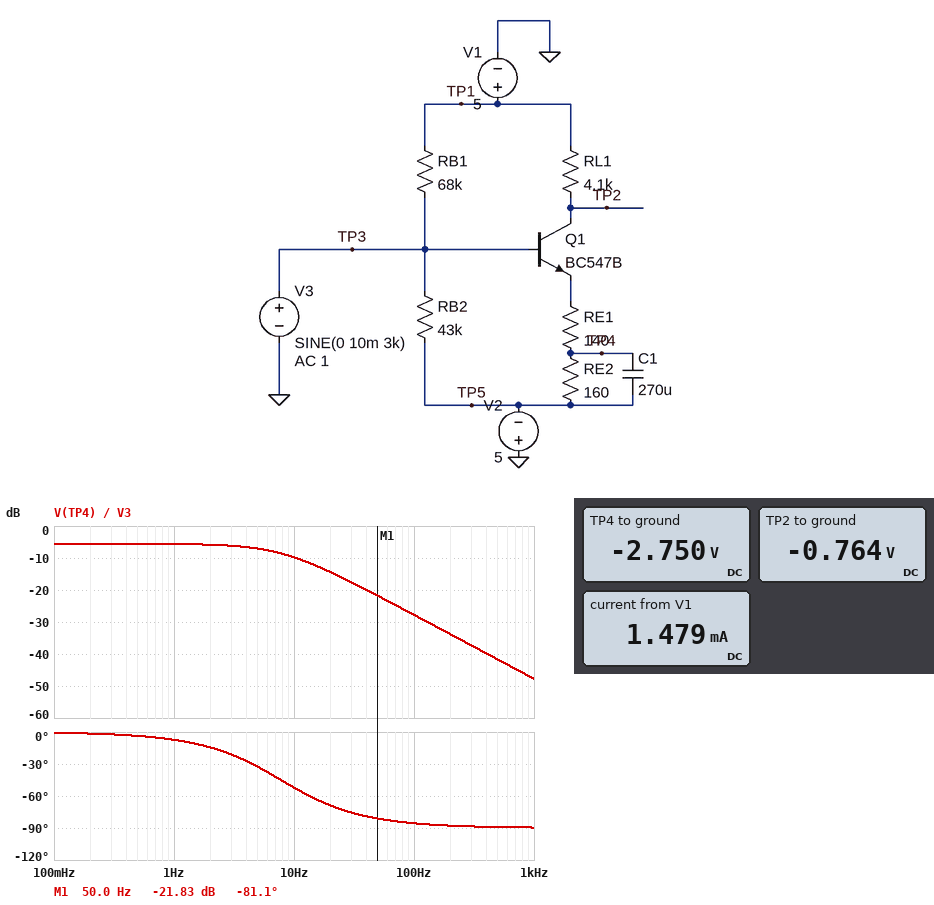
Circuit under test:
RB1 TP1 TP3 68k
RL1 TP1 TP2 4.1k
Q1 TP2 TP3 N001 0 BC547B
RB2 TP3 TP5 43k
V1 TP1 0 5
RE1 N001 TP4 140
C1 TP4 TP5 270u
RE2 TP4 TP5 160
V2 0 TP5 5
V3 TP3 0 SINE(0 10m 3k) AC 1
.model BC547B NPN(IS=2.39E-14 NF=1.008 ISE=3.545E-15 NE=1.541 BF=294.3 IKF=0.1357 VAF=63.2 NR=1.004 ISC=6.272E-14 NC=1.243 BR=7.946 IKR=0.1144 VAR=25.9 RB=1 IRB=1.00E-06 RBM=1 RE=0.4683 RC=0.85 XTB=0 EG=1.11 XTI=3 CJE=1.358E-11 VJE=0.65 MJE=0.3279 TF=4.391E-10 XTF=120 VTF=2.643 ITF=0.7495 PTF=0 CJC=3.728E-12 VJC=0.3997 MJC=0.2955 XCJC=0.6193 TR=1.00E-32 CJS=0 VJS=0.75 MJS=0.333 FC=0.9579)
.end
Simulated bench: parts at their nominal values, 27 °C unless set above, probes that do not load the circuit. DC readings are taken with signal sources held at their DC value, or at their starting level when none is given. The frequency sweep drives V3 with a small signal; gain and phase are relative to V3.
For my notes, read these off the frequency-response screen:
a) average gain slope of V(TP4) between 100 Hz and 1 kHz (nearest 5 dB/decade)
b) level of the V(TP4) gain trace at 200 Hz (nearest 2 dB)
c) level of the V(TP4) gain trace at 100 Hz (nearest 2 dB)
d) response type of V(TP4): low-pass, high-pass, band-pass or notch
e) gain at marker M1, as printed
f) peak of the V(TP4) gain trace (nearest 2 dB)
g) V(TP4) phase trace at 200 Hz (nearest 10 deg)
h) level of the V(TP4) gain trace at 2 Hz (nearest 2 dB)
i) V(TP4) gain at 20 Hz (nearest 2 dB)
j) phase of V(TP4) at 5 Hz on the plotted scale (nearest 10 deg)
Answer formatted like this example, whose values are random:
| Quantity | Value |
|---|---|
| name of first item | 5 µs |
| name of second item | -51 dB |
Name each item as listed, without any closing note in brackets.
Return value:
| Quantity | Value |
|---|---|
| average gain slope of V(TP4) between 100 Hz and 1 kHz | -20 dB/decade |
| level of the V(TP4) gain trace at 200 Hz | -34 dB |
| level of the V(TP4) gain trace at 100 Hz | -28 dB |
| response type of V(TP4): low-pass, high-pass, band-pass or notch | low-pass |
| gain at marker M1, as printed | -21.83 dB |
| peak of the V(TP4) gain trace | -6 dB |
| V(TP4) phase trace at 200 Hz | -90 deg |
| level of the V(TP4) gain trace at 2 Hz | -6 dB |
| V(TP4) gain at 20 Hz | -14 dB |
| phase of V(TP4) at 5 Hz on the plotted scale | -30 deg |
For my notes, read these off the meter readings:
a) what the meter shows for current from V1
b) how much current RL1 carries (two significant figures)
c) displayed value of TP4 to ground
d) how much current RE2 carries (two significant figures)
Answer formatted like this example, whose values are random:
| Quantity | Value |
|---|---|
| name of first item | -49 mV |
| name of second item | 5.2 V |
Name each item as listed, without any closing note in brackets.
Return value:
| Quantity | Value |
|---|---|
| what the meter shows for current from V1 | 1.479 mA |
| how much current RL1 carries | 1.4 mA |
| displayed value of TP4 to ground | -2.750 V |
| how much current RE2 carries | 14 mA |
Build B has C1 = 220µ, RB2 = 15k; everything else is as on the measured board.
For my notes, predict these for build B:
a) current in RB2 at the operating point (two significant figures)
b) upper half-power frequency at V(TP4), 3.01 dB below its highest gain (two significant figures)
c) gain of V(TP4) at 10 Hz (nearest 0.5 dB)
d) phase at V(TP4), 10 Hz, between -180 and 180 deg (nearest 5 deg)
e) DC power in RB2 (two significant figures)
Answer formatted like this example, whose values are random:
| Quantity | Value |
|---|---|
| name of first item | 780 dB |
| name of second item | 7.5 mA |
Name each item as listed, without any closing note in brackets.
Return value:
| Quantity | Value |
|---|---|
| current in RB2 at the operating point | 330 µA |
| upper half-power frequency at V(TP4), 3.01 dB below its highest gain | 9.6 Hz |
| gain of V(TP4) at 10 Hz | -9.0 dB |
| phase at V(TP4), 10 Hz, between -180 and 180 deg | -45 deg |
| DC power in RB2 | 1.7 mW |
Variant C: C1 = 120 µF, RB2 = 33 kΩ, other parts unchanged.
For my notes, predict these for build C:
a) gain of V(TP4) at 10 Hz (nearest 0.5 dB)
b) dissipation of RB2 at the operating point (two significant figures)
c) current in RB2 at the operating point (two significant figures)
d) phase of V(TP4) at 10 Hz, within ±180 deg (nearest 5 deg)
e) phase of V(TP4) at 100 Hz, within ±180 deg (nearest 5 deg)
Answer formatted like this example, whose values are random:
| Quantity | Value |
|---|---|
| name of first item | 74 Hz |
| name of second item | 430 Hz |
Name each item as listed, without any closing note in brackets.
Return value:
| Quantity | Value |
|---|---|
| gain of V(TP4) at 10 Hz | -7.0 dB |
| dissipation of RB2 at the operating point | 760 µW |
| current in RB2 at the operating point | 150 µA |
| phase of V(TP4) at 10 Hz, within ±180 deg | -30 deg |
| phase of V(TP4) at 100 Hz, within ±180 deg | -80 deg |
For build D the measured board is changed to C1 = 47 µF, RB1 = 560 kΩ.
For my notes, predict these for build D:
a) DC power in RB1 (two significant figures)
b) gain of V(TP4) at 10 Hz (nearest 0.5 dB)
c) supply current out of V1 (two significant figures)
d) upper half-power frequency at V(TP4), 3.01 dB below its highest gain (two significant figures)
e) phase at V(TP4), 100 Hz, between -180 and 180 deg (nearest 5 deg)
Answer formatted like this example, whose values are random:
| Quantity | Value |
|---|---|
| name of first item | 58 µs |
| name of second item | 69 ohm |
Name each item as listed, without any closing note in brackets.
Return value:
| Quantity | Value |
|---|---|
| DC power in RB1 | 45 µW |
| gain of V(TP4) at 10 Hz | -6.0 dB |
| supply current out of V1 | 1.4 mA |
| upper half-power frequency at V(TP4), 3.01 dB below its highest gain | 45 Hz |
| phase at V(TP4), 100 Hz, between -180 and 180 deg | -65 deg |
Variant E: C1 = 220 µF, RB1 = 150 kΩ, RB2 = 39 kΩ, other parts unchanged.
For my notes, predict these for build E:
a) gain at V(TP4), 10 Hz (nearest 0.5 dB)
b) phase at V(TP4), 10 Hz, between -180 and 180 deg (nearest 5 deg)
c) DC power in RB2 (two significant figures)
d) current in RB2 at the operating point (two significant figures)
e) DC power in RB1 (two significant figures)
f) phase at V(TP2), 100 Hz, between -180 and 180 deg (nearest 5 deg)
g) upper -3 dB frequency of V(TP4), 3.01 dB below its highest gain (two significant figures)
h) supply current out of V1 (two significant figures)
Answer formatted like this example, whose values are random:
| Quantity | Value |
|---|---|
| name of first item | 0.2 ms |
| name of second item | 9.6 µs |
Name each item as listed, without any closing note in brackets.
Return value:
| Quantity | Value |
|---|---|
| gain at V(TP4), 10 Hz | -9.0 dB |
| phase at V(TP4), 10 Hz, between -180 and 180 deg | -45 deg |
| DC power in RB2 | 640 µW |
| current in RB2 at the operating point | 130 µA |
| DC power in RB1 | 170 µW |
| phase at V(TP2), 100 Hz, between -180 and 180 deg | 0 deg |
| upper -3 dB frequency of V(TP4), 3.01 dB below its highest gain | 9.6 Hz |
| supply current out of V1 | 1.4 mA |
